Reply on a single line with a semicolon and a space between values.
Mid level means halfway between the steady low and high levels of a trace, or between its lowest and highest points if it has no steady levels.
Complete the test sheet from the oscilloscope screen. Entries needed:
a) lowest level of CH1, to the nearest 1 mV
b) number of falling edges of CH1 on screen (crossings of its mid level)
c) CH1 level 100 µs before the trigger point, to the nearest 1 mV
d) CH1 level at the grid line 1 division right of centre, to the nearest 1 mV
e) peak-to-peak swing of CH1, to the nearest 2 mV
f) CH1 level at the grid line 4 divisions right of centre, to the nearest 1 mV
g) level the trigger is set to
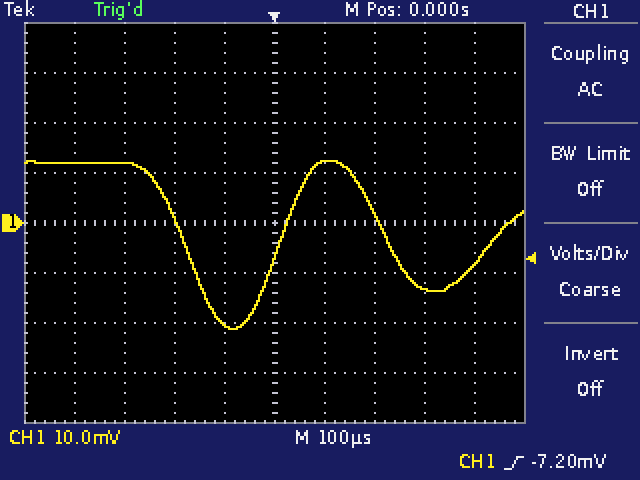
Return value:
-21 mV; 2; -20 mV; 12 mV; 34 mV; -8 mV; -7.20 mV
